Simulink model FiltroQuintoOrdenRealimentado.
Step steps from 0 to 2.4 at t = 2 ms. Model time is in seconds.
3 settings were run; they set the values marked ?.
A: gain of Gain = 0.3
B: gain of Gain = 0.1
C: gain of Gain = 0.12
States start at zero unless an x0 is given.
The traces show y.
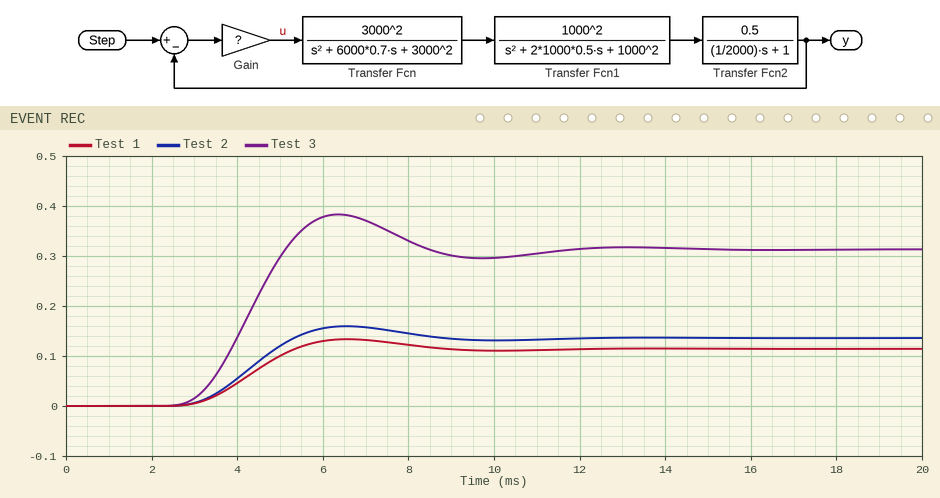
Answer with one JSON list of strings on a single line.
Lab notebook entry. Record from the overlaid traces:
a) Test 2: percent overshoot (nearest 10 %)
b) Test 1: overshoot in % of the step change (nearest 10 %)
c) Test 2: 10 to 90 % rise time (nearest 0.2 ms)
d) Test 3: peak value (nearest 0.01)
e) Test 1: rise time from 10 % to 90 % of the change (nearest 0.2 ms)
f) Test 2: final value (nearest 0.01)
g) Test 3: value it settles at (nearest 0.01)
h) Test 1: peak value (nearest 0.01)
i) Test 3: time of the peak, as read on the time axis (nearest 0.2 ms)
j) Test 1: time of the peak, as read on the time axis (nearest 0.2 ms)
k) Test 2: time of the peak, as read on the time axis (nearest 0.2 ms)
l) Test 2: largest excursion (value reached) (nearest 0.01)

["20 %", "20 %", "1.8 ms", "0.38", "1.8 ms", "0.14", "0.31", "0.13", "6.4 ms", "6.6 ms", "6.6 ms", "0.16"]
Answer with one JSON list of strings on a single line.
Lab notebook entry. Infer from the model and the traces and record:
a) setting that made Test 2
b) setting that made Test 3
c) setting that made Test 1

["C", "A", "B"]
